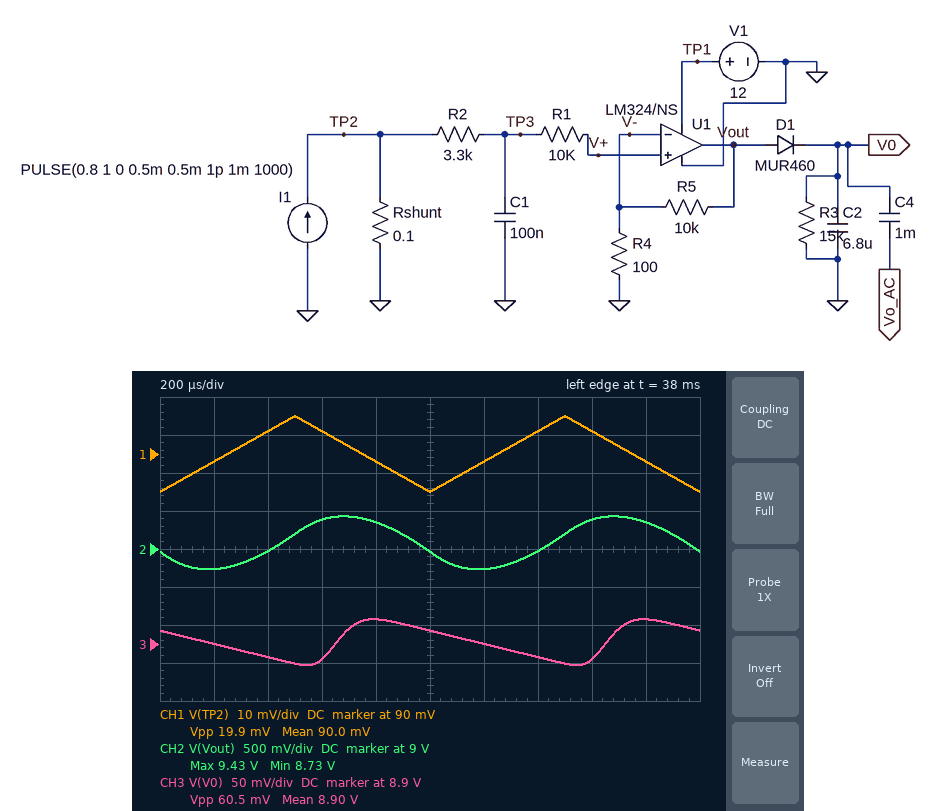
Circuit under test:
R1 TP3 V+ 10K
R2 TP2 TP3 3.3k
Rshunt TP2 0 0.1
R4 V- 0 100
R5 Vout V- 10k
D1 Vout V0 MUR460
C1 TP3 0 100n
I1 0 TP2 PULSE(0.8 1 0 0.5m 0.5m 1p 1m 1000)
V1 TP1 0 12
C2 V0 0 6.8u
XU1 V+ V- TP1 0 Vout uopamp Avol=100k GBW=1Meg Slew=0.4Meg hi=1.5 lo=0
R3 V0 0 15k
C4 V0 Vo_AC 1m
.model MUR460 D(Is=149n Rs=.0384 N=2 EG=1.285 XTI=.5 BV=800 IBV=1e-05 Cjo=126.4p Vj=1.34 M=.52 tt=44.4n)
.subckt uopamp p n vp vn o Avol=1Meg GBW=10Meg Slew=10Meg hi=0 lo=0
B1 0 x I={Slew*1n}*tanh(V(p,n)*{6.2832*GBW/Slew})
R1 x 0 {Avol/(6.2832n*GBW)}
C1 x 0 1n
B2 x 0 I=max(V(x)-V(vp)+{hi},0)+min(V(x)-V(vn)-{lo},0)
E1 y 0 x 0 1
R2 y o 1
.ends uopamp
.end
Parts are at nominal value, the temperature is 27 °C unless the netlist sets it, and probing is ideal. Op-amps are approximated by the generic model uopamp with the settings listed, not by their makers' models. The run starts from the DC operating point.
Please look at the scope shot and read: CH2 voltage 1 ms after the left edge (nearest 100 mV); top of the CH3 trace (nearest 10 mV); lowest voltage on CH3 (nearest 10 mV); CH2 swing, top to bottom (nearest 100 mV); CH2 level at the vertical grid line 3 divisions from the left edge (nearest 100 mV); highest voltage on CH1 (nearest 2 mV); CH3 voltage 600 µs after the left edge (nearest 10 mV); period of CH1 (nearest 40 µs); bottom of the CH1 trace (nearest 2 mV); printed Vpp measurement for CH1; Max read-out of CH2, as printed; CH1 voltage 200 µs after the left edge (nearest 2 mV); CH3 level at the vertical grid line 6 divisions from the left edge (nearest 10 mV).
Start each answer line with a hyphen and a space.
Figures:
- 9.0 V
- 8.93 V
- 8.87 V
- 700 mV
- 9.4 V
- 100 mV
- 8.88 V
- 1.00 ms
- 80 mV
- 19.9 mV
- 9.43 V
- 88 mV
- 8.90 V
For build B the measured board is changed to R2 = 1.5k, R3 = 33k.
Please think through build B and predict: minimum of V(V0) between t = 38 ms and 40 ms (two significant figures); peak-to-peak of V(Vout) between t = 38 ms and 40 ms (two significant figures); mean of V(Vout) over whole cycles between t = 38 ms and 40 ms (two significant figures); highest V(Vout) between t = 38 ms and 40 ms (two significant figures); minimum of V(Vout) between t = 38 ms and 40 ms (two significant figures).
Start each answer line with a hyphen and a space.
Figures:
- 9.2 V
- 1.2 V
- 9.1 V
- 9.7 V
- 8.5 V
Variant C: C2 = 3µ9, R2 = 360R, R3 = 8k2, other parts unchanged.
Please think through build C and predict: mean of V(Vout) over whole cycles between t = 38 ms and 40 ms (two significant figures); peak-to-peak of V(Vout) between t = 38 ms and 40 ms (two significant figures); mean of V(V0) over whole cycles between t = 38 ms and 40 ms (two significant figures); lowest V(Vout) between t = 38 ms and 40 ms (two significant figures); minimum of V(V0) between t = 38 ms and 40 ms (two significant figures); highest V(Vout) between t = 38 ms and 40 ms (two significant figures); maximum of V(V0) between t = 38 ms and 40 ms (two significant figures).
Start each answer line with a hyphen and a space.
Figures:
- 9.1 V
- 1.8 V
- 9.3 V
- 8.2 V
- 9.2 V
- 10 V
- 9.4 V
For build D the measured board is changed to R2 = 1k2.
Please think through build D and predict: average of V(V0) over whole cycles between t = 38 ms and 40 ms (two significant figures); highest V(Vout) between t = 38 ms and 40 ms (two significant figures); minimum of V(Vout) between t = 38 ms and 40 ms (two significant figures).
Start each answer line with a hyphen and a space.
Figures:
- 9.2 V
- 9.8 V
- 8.4 V
